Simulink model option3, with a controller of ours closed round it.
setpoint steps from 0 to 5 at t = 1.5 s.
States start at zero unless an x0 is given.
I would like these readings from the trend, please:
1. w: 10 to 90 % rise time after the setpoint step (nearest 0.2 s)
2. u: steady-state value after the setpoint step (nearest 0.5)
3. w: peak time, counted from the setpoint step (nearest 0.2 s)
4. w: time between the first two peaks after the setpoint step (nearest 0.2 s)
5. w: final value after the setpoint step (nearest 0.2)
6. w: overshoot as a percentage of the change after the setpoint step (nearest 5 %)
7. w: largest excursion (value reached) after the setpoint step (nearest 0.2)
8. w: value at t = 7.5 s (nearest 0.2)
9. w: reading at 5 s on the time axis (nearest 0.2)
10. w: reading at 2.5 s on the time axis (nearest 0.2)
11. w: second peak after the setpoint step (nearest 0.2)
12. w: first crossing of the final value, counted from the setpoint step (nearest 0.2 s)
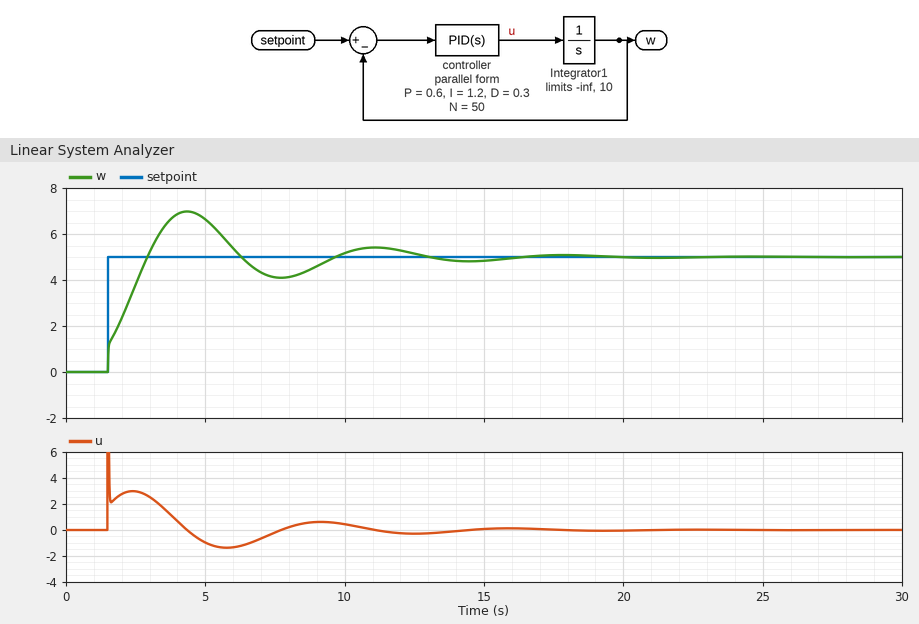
1.2 s
0.0
2.8 s
6.8 s
5.0
40 %
7.0
4.2
6.6
3.8
5.4
1.4 s
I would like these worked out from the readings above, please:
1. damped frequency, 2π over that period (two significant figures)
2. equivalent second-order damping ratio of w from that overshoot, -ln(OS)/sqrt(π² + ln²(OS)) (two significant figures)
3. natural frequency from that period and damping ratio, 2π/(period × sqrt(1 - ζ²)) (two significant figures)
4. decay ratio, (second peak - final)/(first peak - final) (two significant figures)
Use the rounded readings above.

0.92 rad/s
0.28
0.96 rad/s
0.20
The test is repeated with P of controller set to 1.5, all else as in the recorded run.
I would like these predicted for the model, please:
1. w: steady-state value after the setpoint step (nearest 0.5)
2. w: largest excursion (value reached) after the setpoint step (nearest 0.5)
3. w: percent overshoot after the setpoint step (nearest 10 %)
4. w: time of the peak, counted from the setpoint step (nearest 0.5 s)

5.0
6.0
20 %
2.5 s
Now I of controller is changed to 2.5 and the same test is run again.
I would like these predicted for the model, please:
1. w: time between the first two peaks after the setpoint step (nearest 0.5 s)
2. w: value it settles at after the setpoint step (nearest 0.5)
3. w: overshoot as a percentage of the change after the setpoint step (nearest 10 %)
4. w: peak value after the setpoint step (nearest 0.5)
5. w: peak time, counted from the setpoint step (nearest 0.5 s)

4.5 s
5.0
50 %
7.5
2.0 s
